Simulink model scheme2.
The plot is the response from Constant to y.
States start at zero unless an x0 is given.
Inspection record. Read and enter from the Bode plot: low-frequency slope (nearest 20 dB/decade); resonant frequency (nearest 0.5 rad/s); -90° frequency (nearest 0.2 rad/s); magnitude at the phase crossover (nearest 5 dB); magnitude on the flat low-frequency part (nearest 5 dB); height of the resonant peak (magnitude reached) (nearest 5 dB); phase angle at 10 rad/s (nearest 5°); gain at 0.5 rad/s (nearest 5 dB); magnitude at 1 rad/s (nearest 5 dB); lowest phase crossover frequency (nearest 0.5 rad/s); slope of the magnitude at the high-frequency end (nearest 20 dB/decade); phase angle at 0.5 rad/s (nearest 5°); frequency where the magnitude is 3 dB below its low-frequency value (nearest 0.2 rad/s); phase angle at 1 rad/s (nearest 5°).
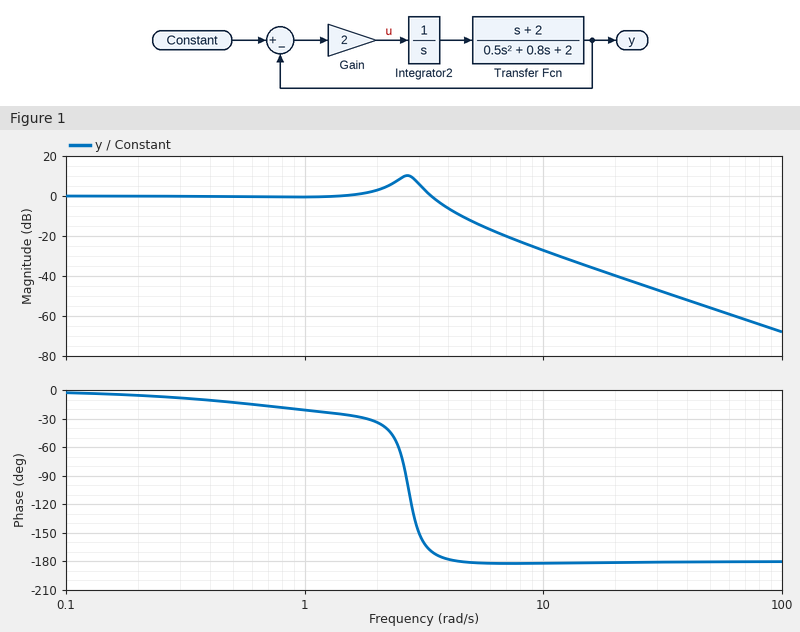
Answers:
0 dB/decade
2.5 rad/s
2.6 rad/s
-10 dB
0 dB
10 dB
-180°
0 dB
0 dB
4.5 rad/s
-40 dB/decade
-15°
3.6 rad/s
-20°
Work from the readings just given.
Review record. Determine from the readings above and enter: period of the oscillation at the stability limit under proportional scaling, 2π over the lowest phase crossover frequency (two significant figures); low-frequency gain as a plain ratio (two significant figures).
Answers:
1.4 s
1.0
